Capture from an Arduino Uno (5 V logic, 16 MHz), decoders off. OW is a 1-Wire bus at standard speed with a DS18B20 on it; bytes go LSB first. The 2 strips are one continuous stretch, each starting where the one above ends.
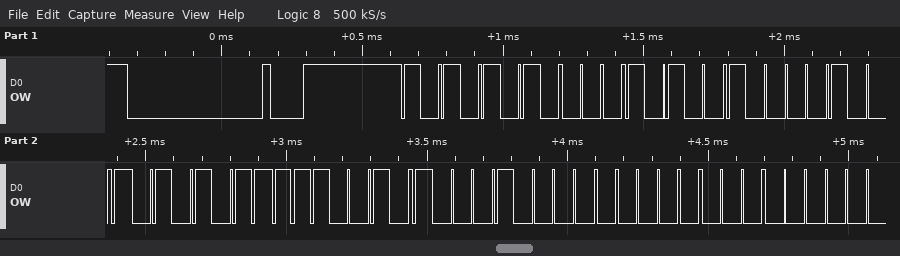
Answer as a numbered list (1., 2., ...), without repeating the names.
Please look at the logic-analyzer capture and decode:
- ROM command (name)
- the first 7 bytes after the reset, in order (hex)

1. Match ROM
2. 55 28 21 D5 A7 08 00
